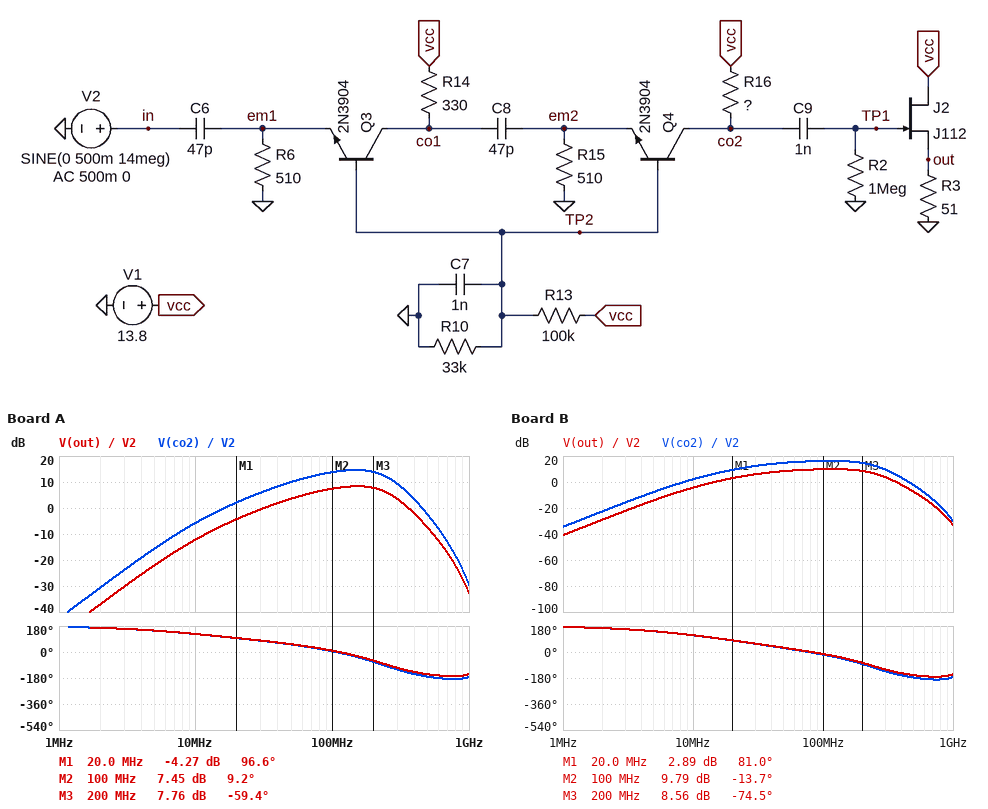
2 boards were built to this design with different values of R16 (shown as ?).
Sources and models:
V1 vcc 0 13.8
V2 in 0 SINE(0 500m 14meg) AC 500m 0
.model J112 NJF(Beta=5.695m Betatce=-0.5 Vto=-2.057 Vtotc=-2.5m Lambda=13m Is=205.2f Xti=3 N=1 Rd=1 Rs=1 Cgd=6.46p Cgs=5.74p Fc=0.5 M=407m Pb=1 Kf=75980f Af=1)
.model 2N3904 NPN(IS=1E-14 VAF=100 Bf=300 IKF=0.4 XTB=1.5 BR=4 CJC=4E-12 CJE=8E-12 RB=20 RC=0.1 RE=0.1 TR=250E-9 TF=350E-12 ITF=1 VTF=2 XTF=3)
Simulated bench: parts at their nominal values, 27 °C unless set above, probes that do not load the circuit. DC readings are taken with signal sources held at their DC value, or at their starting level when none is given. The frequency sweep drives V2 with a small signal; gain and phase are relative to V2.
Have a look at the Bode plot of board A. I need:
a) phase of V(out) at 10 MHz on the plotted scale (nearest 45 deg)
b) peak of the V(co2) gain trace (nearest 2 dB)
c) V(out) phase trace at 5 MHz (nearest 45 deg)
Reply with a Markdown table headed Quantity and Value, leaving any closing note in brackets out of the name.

| Quantity | Value |
|---|---|
| phase of V(out) at 10 MHz on the plotted scale | 135 deg |
| peak of the V(co2) gain trace | 14 dB |
| V(out) phase trace at 5 MHz | 135 deg |
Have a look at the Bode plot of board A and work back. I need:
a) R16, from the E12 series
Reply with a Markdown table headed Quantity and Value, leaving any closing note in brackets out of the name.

| Quantity | Value |
|---|---|
| R16, from the E12 series | 270 Ω |
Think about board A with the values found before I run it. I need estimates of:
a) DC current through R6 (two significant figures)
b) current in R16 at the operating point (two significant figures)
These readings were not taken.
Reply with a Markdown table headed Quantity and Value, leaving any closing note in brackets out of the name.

| Quantity | Value |
|---|---|
| DC current through R6 | 4.1 mA |
| current in R16 at the operating point | 4.1 mA |
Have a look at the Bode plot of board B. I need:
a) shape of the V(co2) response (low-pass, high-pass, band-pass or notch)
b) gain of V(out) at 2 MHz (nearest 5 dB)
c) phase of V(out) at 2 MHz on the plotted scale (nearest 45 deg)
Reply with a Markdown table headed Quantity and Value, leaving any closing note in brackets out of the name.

| Quantity | Value |
|---|---|
| shape of the V(co2) response | band-pass |
| gain of V(out) at 2 MHz | -30 dB |
| phase of V(out) at 2 MHz on the plotted scale | 180 deg |
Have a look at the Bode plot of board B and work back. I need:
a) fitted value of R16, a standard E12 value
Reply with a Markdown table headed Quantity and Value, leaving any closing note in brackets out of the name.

| Quantity | Value |
|---|---|
| fitted value of R16, a standard E12 value | 680 Ω |
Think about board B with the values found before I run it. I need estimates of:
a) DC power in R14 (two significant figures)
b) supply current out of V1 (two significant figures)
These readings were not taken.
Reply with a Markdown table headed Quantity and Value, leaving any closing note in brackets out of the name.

| Quantity | Value |
|---|---|
| DC power in R14 | 5.6 mW |
| supply current out of V1 | 21 mA |
